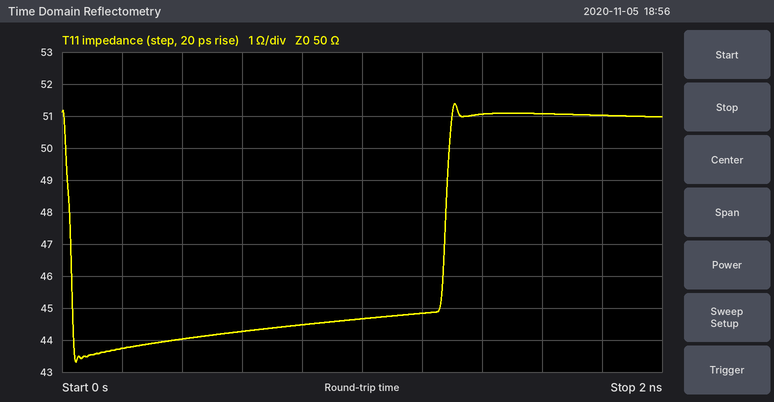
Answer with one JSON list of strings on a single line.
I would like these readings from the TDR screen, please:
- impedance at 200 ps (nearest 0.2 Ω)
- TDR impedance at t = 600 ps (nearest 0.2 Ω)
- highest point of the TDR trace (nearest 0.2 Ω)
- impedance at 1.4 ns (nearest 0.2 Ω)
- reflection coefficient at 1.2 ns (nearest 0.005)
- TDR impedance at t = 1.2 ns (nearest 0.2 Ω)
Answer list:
["43.8 Ω", "44.2 Ω", "51.4 Ω", "51.0 Ω", "-0.055", "44.8 Ω"]
